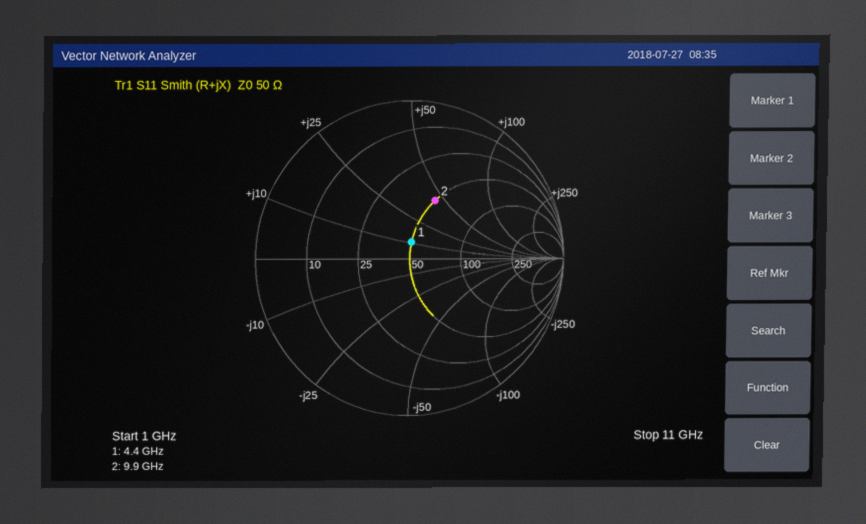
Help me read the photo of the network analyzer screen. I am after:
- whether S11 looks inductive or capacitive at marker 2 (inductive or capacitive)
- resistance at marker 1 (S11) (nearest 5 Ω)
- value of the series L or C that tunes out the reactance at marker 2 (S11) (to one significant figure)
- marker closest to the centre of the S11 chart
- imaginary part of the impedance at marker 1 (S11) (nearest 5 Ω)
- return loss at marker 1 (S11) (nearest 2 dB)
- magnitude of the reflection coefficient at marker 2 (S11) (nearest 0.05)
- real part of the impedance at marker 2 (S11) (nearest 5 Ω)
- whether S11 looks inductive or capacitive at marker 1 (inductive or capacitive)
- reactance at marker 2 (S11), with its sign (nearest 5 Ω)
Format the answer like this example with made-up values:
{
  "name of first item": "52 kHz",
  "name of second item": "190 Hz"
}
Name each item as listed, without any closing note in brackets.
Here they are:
{
  "whether S11 looks inductive or capacitive at marker 2": "inductive",
  "resistance at marker 1 (S11)": "50 Ω",
  "value of the series L or C that tunes out the reactance at marker 2 (S11)": "400 fF",
  "marker closest to the centre of the S11 chart": "marker 1",
  "imaginary part of the impedance at marker 1 (S11)": "+10 Ω",
  "return loss at marker 1 (S11)": "20 dB",
  "magnitude of the reflection coefficient at marker 2 (S11)": "0.40",
  "real part of the impedance at marker 2 (S11)": "50 Ω",
  "whether S11 looks inductive or capacitive at marker 1": "inductive",
  "reactance at marker 2 (S11), with its sign": "+45 Ω"
}
